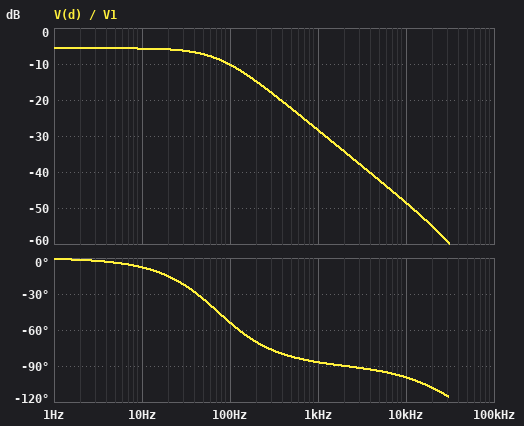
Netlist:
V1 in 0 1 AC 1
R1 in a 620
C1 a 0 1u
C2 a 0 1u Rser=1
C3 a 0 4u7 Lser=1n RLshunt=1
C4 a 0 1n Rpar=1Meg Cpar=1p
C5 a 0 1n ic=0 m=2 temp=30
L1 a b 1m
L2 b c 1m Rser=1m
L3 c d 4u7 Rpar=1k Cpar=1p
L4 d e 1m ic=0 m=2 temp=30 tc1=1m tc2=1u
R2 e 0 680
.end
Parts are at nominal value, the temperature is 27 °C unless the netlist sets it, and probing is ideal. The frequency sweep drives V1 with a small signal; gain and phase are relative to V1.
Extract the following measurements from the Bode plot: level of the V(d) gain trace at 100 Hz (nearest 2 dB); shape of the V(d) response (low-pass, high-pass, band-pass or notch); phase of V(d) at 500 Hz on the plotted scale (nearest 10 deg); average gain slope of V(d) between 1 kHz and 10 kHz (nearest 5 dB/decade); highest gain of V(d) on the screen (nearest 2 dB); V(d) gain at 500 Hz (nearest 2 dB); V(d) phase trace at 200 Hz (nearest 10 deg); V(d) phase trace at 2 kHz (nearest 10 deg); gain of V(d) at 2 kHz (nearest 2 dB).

-10 dB
low-pass
-80 deg
-20 dB/decade
-6 dB
-22 dB
-70 deg
-90 deg
-34 dB
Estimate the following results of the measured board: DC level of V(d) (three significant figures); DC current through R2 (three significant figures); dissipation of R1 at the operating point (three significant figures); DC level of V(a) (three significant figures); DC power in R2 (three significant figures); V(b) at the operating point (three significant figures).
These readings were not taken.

523 mV
769 µA
367 µW
523 mV
402 µW
523 mV
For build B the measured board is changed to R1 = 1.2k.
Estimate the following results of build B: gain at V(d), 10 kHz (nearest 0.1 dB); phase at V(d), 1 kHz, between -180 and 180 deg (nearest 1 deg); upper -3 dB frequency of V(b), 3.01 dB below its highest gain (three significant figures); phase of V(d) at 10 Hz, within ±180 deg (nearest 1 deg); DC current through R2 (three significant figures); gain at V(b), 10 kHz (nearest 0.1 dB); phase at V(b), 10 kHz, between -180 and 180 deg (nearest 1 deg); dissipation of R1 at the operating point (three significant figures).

-54.3 dB
-88 deg
54.8 Hz
-10 deg
532 µA
-54.2 dB
-94 deg
340 µW
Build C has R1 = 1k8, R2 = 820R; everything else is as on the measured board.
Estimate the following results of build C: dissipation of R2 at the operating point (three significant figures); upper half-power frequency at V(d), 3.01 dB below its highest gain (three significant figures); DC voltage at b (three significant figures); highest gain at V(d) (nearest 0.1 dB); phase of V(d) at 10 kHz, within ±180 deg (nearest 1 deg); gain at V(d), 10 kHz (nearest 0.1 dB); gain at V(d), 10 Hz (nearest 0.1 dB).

119 µW
42.2 Hz
313 mV
-10.1 dB
-98 deg
-57.7 dB
-10.3 dB
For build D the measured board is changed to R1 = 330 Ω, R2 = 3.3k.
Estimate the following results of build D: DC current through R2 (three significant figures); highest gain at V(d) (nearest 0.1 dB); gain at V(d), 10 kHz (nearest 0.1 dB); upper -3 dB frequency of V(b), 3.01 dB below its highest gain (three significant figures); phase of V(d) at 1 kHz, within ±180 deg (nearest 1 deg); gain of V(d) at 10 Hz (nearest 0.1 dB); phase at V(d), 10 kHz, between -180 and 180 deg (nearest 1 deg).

275 µA
-0.8 dB
-42.9 dB
79.2 Hz
-86 deg
-0.9 dB
-91 deg
